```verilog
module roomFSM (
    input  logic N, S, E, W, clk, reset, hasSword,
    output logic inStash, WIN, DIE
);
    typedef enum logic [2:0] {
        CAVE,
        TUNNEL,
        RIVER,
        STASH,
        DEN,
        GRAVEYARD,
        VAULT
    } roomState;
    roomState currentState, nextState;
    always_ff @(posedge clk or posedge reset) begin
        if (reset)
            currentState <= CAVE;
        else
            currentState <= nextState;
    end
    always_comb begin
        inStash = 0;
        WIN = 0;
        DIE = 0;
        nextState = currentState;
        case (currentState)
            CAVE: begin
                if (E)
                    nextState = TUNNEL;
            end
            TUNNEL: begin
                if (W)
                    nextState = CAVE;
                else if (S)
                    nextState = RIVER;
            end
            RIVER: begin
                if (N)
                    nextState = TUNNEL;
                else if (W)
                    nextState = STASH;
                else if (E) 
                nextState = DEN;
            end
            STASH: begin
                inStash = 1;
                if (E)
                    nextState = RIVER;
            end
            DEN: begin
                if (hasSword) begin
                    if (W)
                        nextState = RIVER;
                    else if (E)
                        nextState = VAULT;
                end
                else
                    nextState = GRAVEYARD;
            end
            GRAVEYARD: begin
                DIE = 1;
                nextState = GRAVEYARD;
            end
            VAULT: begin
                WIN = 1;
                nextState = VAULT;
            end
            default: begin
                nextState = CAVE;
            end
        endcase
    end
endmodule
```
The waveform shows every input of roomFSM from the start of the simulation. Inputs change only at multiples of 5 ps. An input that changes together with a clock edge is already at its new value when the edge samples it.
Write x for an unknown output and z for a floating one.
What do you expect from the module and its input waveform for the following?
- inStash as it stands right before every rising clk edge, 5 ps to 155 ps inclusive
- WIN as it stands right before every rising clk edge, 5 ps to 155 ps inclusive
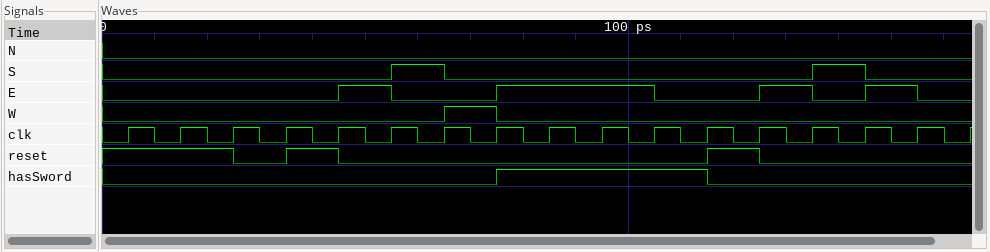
0 0 0 0 0 0 0 1 0 0 0 0 0 0 0 0
0 0 0 0 0 0 0 0 0 0 1 1 0 0 0 0
